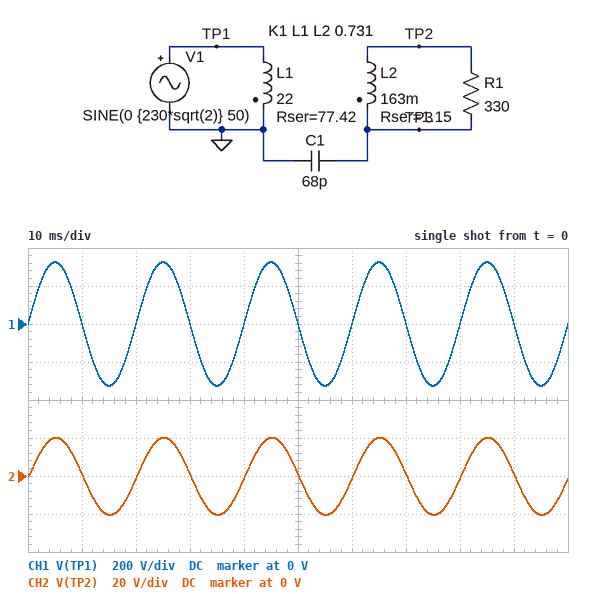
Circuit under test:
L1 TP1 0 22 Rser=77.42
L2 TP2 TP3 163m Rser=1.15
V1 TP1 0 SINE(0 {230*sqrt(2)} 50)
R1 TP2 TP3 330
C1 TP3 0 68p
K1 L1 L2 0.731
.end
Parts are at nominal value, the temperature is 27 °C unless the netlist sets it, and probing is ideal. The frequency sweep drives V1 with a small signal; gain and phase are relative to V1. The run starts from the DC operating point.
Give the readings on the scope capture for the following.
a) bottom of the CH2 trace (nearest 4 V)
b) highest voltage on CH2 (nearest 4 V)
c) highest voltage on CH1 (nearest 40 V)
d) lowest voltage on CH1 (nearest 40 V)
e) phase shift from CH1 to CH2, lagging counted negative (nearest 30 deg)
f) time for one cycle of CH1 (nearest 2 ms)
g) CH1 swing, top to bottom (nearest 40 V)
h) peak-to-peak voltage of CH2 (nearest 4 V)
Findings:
-20 V
20 V
320 V
-320 V
0 deg
20 ms
640 V
40 V
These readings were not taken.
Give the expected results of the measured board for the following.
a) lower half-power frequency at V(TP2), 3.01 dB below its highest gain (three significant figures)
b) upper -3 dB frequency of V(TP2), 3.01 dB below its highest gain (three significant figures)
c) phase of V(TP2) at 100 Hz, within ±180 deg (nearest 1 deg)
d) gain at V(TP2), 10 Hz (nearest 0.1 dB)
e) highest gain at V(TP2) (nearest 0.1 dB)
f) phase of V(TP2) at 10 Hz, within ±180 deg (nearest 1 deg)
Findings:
559 mHz
696 Hz
-8 deg
-24.1 dB
-24.1 dB
2 deg
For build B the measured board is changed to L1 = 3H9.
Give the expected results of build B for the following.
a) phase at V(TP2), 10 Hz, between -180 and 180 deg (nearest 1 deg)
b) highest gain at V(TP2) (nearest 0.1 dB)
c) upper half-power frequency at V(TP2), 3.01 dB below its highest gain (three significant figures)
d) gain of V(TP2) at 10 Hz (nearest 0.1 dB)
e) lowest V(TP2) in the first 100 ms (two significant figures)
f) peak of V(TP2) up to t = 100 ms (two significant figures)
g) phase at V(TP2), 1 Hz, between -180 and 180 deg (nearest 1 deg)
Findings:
17 deg
-16.6 dB
704 Hz
-17.0 dB
-50 V
47 V
72 deg
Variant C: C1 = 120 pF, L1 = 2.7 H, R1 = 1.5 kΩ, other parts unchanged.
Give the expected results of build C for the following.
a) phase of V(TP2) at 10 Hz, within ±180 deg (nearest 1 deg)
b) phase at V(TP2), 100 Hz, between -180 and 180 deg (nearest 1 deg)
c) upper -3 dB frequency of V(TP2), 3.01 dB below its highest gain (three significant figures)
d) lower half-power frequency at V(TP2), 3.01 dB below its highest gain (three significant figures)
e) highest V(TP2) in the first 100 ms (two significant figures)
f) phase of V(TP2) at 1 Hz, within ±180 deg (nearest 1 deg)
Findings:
24 deg
1 deg
3.16 kHz
4.54 Hz
58 V
78 deg
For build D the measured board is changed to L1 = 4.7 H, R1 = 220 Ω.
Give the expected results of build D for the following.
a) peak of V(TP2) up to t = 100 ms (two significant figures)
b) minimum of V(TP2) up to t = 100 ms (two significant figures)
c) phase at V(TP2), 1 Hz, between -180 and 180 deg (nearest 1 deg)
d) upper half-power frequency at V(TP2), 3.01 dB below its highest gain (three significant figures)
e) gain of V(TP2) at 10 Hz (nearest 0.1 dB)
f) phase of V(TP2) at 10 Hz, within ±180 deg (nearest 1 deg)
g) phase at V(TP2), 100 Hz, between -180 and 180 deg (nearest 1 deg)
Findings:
43 V
-45 V
69 deg
472 Hz
-17.7 dB
13 deg
-11 deg
